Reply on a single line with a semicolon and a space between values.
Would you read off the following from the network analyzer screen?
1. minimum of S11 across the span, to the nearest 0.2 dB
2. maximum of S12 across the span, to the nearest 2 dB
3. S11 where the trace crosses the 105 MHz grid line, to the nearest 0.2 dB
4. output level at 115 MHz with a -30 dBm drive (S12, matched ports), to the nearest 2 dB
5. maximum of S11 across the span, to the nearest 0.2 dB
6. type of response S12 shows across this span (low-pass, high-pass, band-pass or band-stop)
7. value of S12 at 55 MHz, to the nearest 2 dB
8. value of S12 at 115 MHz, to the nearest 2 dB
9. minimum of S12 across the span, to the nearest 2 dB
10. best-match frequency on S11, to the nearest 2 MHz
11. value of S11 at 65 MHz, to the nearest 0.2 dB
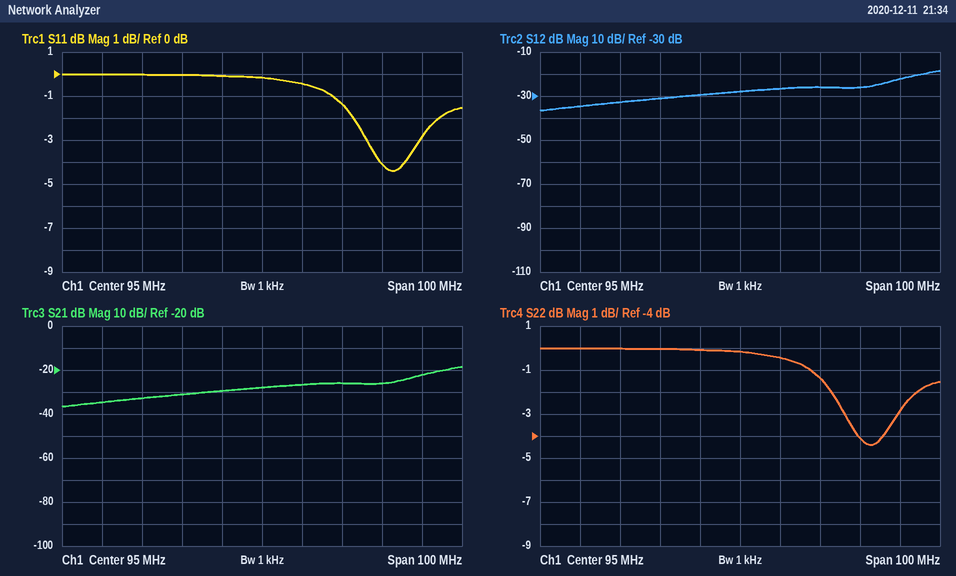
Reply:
-4.4 dB; -18 dB; -0.4 dB; -56 dBm; 0.0 dB; high-pass; -34 dB; -26 dB; -36 dB; 128 MHz; 0.0 dB
